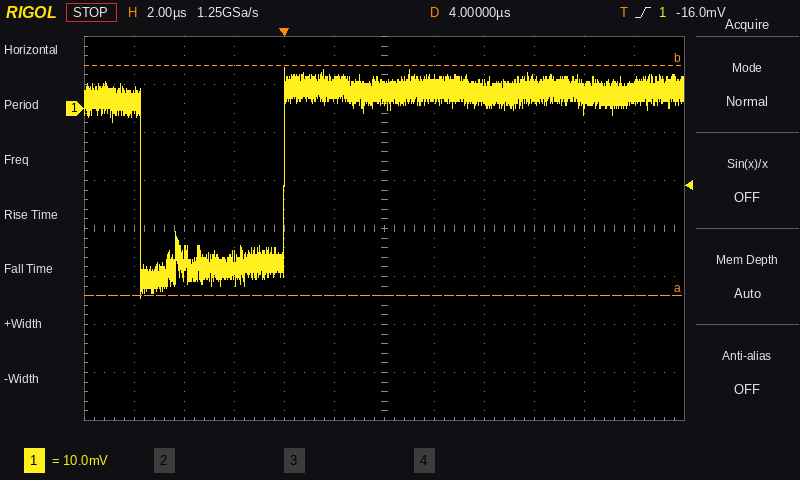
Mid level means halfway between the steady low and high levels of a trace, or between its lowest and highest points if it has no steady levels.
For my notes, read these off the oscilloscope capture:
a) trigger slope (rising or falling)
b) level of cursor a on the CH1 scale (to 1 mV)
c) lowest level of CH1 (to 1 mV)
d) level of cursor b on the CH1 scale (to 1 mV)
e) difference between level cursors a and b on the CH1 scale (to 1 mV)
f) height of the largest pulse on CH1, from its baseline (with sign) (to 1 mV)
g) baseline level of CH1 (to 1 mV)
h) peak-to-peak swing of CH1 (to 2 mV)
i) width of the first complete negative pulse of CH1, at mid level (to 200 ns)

rising
-39 mV
-39 mV
9 mV
48 mV
-43 mV
4 mV
48 mV
5.8 µs
